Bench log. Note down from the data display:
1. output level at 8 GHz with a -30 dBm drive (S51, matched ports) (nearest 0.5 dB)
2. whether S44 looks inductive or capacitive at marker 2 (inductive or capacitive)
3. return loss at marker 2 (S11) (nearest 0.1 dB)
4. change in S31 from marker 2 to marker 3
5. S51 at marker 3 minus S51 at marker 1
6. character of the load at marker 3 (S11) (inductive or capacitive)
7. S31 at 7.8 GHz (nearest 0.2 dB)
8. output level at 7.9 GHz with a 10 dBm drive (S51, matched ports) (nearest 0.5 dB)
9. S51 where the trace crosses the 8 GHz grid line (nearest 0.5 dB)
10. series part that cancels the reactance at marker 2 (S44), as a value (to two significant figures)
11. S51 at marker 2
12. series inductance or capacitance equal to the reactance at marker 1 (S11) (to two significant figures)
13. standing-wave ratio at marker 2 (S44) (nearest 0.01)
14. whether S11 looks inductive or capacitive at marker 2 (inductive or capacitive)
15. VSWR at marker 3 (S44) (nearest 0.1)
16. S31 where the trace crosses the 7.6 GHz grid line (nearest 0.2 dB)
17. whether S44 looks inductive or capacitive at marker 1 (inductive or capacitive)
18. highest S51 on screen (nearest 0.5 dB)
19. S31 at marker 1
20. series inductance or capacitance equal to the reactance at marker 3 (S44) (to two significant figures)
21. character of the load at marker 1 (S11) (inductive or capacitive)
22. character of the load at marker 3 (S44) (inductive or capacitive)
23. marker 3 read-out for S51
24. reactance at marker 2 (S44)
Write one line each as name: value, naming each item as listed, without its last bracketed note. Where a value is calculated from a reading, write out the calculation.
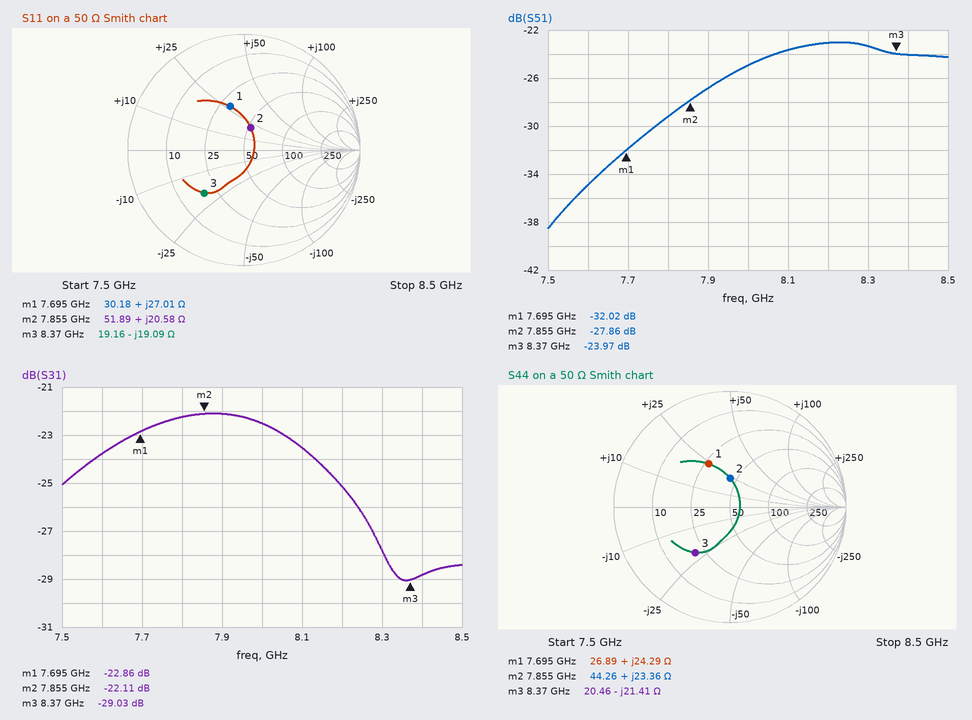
output level at 8 GHz with a -30 dBm drive (S51, matched ports): -30 dBm + (-25.0 dB) = -55.0 dBm
whether S44 looks inductive or capacitive at marker 2: inductive
return loss at marker 2 (S11): 14.0 dB
change in S31 from marker 2 to marker 3: -29.03 − (-22.11) = -6.92 dB
S51 at marker 3 minus S51 at marker 1: -23.97 − (-32.02) = 8.05 dB
character of the load at marker 3 (S11): capacitive
S31 at 7.8 GHz: -22.2 dB
output level at 7.9 GHz with a 10 dBm drive (S51, matched ports): 10 dBm + (-27.0 dB) = -17.0 dBm
S51 where the trace crosses the 8 GHz grid line: -25.0 dB
series part that cancels the reactance at marker 2 (S44), as a value: C = 1/(2π × 7.855 GHz × 23.36 Ω) ≈ 867 fF, so 870 fF to two significant figures
S51 at marker 2: -27.86 dB
series inductance or capacitance equal to the reactance at marker 1 (S11): L = 27.01 Ω/(2π × 7.695 GHz) ≈ 559 pH, so 560 pH to two significant figures
standing-wave ratio at marker 2 (S44): 1.66
whether S11 looks inductive or capacitive at marker 2: inductive
VSWR at marker 3 (S44): 3.0
S31 where the trace crosses the 7.6 GHz grid line: -23.8 dB
whether S44 looks inductive or capacitive at marker 1: inductive
highest S51 on screen: -23.0 dB
S31 at marker 1: -22.86 dB
series inductance or capacitance equal to the reactance at marker 3 (S44): C = 1/(2π × 8.37 GHz × 21.41 Ω) ≈ 888 fF, so 890 fF to two significant figures
character of the load at marker 1 (S11): inductive
character of the load at marker 3 (S44): capacitive
marker 3 read-out for S51: -23.97 dB
reactance at marker 2: +23.36 Ω
